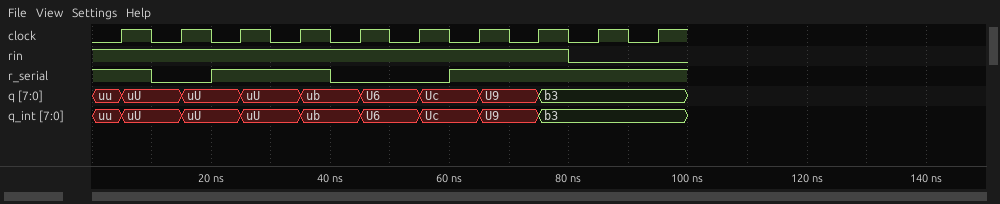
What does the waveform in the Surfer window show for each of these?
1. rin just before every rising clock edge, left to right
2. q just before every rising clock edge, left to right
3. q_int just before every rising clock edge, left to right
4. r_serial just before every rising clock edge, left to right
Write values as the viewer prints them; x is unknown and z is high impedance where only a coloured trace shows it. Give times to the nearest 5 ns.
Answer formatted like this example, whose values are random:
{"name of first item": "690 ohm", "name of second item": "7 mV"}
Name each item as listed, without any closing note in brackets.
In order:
{"rin just before every rising clock edge, left to right": "1 1 1 1 1 1 1 1 0 0", "q just before every rising clock edge, left to right": "uu, uU, uU, uU, ub, U6, Uc, U9, b3, b3", "q_int just before every rising clock edge, left to right": "uu, uU, uU, uU, ub, U6, Uc, U9, b3, b3", "r_serial just before every rising clock edge, left to right": "1 0 1 1 0 0 1 1 1 1"}
